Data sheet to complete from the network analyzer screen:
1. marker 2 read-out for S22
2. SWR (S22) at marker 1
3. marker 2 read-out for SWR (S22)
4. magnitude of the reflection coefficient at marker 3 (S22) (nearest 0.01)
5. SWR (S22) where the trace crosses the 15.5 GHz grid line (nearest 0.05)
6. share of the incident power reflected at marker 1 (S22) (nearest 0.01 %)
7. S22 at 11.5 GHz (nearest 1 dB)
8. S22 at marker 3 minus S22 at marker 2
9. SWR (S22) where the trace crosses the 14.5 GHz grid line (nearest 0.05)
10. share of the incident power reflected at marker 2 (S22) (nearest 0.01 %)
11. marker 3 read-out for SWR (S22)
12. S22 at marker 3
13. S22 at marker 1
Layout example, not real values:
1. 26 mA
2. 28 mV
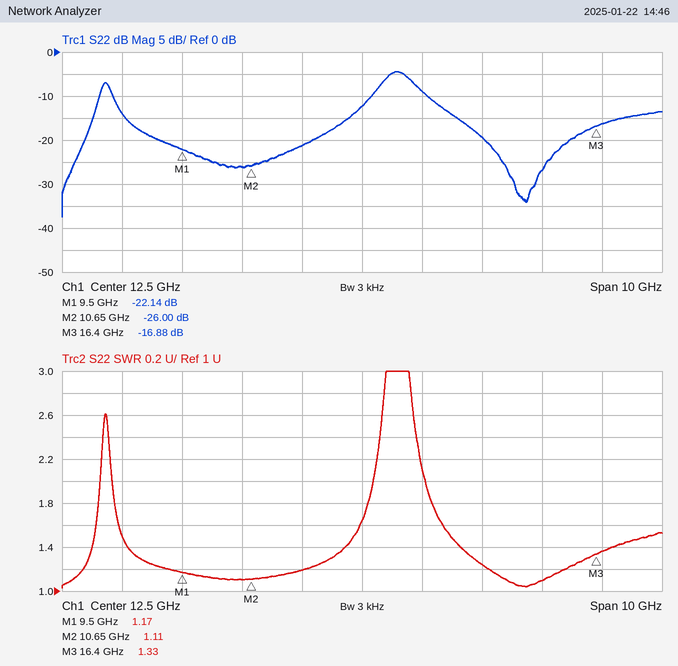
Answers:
1. -26.00 dB
2. 1.17
3. 1.11
4. 0.14
5. 1.10
6. 0.61 %
7. -21 dB
8. 9.12 dB
9. 1.25
10. 0.25 %
11. 1.33
12. -16.88 dB
13. -22.14 dB
